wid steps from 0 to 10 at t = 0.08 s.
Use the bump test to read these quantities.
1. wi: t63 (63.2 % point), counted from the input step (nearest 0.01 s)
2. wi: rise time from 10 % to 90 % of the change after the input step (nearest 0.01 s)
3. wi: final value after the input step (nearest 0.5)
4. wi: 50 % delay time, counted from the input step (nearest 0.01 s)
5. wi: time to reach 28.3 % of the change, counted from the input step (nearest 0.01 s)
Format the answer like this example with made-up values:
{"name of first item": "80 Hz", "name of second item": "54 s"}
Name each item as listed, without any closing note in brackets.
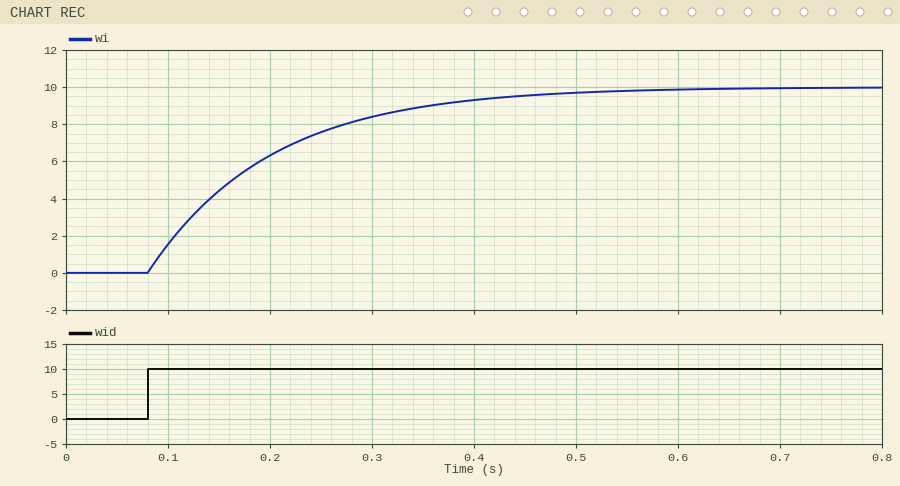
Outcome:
{"wi: t63 (63.2 % point), counted from the input step": "0.12 s", "wi: rise time from 10 % to 90 % of the change after the input step": "0.26 s", "wi: final value after the input step": "10.0", "wi: 50 % delay time, counted from the input step": "0.08 s", "wi: time to reach 28.3 % of the change, counted from the input step": "0.04 s"}
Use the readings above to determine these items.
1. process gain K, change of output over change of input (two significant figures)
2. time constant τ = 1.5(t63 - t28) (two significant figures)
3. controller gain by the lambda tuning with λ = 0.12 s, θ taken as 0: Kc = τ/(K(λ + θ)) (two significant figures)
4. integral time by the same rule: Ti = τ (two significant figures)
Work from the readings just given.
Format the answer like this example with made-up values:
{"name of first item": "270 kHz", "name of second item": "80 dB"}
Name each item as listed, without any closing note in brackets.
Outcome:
{"process gain K, change of output over change of input": "1.0", "time constant τ = 1.5(t63 - t28)": "0.12 s", "controller gain by the lambda tuning with λ = 0.12 s, θ taken as 0: Kc = τ/(K(λ + θ))": "1.0", "integral time by the same rule: Ti = τ": "0.12 s"}
